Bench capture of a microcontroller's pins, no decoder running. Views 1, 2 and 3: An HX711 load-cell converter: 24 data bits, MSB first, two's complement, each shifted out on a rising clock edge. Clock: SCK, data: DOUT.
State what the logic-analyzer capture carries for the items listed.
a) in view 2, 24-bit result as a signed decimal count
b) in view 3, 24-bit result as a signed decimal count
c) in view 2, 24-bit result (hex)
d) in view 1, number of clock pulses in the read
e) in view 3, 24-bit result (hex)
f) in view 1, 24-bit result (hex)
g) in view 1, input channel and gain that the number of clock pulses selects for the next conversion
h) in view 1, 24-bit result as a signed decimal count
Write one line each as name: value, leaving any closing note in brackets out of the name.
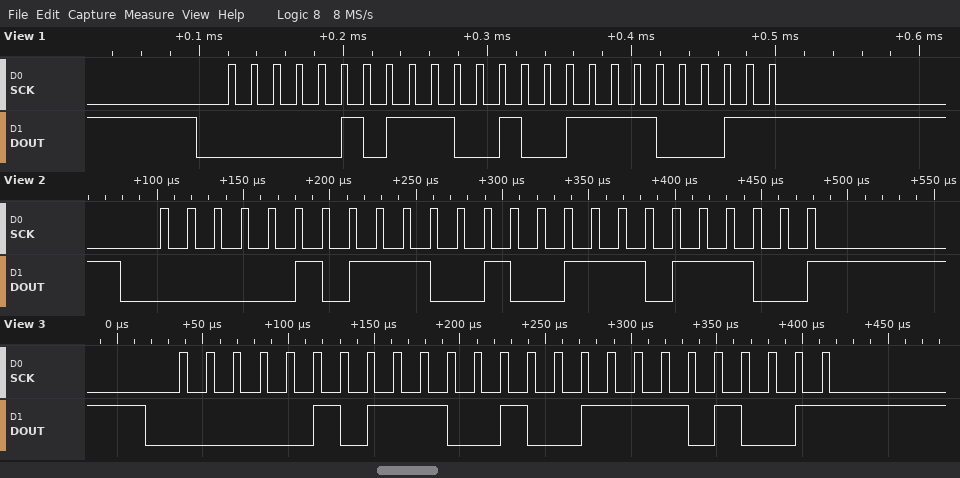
in view 2, 24-bit result as a signed decimal count: 379356
in view 3, 24-bit result as a signed decimal count: 379369
in view 2, 24-bit result: 0x05C9DC
in view 1, number of clock pulses in the read: 25
in view 3, 24-bit result: 0x05C9E9
in view 1, 24-bit result: 0x05C9E3
in view 1, input channel and gain that the number of clock pulses selects for the next conversion: channel A, gain 128
in view 1, 24-bit result as a signed decimal count: 379363
